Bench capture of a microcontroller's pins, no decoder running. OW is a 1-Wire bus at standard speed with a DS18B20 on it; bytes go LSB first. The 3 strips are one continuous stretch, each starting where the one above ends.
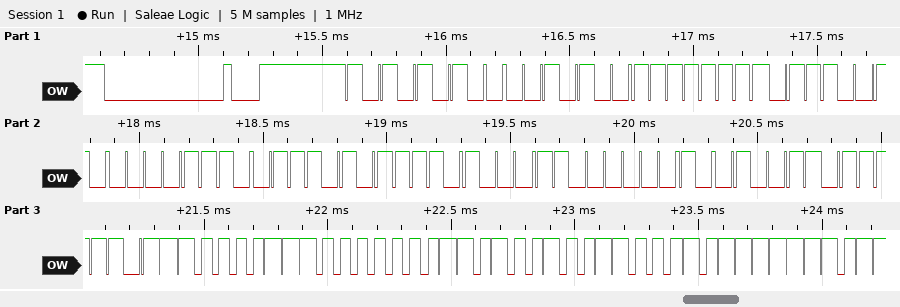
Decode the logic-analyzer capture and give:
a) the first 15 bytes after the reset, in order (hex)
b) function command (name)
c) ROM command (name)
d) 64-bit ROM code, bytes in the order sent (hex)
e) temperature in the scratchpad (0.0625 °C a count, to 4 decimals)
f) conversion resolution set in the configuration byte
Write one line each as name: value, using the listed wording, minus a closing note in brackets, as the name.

the first 15 bytes after the reset, in order: 55 28 FF 4E 70 AE 17 03 C9 BE C3 01 4B 46 7F
function command: Read Scratchpad
ROM command: Match ROM
64-bit ROM code, bytes in the order sent: 28 FF 4E 70 AE 17 03 C9
temperature in the scratchpad: 28.1875 °C
conversion resolution set in the configuration byte: 12 bits
